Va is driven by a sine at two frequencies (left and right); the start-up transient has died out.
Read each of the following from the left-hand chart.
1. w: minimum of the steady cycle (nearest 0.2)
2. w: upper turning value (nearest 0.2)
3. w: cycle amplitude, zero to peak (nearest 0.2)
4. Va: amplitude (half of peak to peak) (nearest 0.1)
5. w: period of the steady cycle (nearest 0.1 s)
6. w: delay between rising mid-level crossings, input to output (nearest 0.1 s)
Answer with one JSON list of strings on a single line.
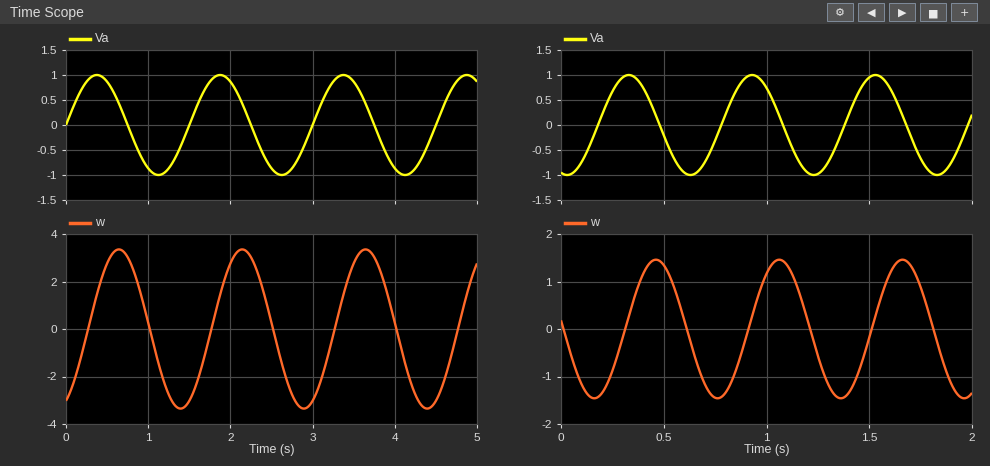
["-3.4", "3.4", "3.4", "1.0", "1.5 s", "0.3 s"]
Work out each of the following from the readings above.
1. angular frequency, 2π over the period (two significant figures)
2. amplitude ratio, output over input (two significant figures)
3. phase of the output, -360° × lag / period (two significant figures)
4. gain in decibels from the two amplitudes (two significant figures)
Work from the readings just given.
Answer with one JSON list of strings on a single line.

["4.2 rad/s", "3.4", "-72°", "11 dB"]
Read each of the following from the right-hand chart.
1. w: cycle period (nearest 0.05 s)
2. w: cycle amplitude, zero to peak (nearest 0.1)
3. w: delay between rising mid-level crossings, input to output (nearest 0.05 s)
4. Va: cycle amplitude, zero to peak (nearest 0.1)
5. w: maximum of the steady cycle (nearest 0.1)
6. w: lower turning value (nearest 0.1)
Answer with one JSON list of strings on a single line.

["0.60 s", "1.5", "0.15 s", "1.0", "1.5", "-1.5"]
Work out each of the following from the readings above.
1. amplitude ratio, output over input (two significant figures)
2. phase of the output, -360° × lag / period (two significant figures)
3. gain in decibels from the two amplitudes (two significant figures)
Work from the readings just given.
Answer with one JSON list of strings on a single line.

["1.5", "-90°", "3.5 dB"]
